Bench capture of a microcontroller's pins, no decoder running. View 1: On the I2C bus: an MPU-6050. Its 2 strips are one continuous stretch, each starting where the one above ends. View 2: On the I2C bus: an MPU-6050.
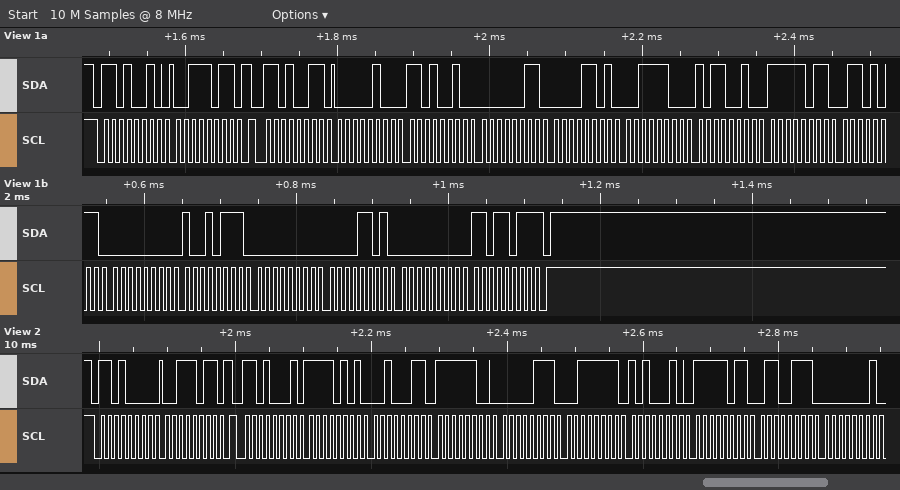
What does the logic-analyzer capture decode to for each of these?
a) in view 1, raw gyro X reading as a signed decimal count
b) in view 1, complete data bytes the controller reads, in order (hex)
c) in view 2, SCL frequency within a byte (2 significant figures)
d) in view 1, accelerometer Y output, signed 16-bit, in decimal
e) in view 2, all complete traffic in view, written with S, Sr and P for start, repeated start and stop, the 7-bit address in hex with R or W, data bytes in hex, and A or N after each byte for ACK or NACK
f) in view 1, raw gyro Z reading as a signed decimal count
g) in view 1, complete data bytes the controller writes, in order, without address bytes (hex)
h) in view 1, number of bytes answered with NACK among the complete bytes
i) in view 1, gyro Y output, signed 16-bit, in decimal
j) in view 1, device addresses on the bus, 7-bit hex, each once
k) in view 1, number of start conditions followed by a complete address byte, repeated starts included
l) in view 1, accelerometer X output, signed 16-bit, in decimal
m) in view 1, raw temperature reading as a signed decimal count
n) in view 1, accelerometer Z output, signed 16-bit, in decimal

151
04 D2 03 0D 3C B2 FB 6B 00 97 00 0D 00 DB
100 kHz
781
S 68W A 3B A Sr 68R A F5 A 23 A FC A 07 A 3F A A2 A FB A 67 A 01 A
219
3B
1
13
0x69
2
1234
-1173
15538
